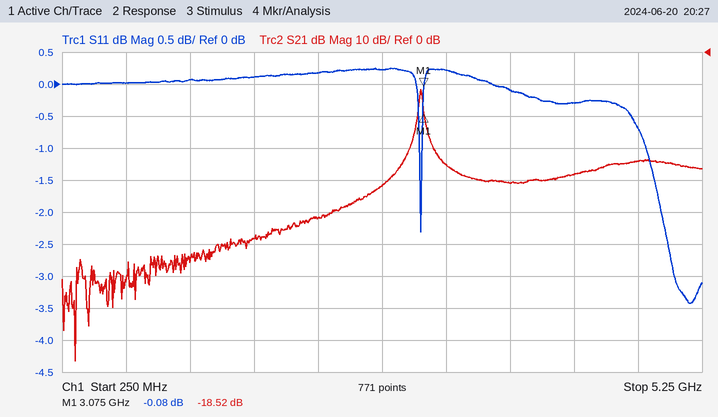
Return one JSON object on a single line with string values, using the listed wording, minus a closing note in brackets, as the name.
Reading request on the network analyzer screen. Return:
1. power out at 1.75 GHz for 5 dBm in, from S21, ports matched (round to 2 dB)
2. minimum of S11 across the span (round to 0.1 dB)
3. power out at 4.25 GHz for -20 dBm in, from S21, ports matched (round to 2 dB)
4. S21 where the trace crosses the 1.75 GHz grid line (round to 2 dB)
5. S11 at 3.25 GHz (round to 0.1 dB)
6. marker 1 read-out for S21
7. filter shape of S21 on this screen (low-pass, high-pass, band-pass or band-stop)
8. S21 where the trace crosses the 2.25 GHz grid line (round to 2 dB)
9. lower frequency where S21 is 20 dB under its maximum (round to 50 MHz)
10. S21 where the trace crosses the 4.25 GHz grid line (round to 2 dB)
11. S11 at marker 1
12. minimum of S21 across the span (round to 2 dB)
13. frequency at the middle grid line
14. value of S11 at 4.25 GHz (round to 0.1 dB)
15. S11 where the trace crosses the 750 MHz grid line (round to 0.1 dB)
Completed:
{"power out at 1.75 GHz for 5 dBm in, from S21, ports matched": "-54 dBm", "minimum of S11 across the span": "-3.4 dB", "power out at 4.25 GHz for -20 dBm in, from S21, ports matched": "-58 dBm", "S21 where the trace crosses the 1.75 GHz grid line": "-58 dB", "S11 at 3.25 GHz": "0.2 dB", "marker 1 read-out for S21": "-18.52 dB", "filter shape of S21 on this screen": "band-pass", "S21 where the trace crosses the 2.25 GHz grid line": "-52 dB", "lower frequency where S21 is 20 dB under its maximum": "2.95 GHz", "S21 where the trace crosses the 4.25 GHz grid line": "-38 dB", "S11 at marker 1": "-0.08 dB", "minimum of S21 across the span": "-96 dB", "frequency at the middle grid line": "2.75 GHz", "value of S11 at 4.25 GHz": "-0.3 dB", "S11 where the trace crosses the 750 MHz grid line": "0.0 dB"}
